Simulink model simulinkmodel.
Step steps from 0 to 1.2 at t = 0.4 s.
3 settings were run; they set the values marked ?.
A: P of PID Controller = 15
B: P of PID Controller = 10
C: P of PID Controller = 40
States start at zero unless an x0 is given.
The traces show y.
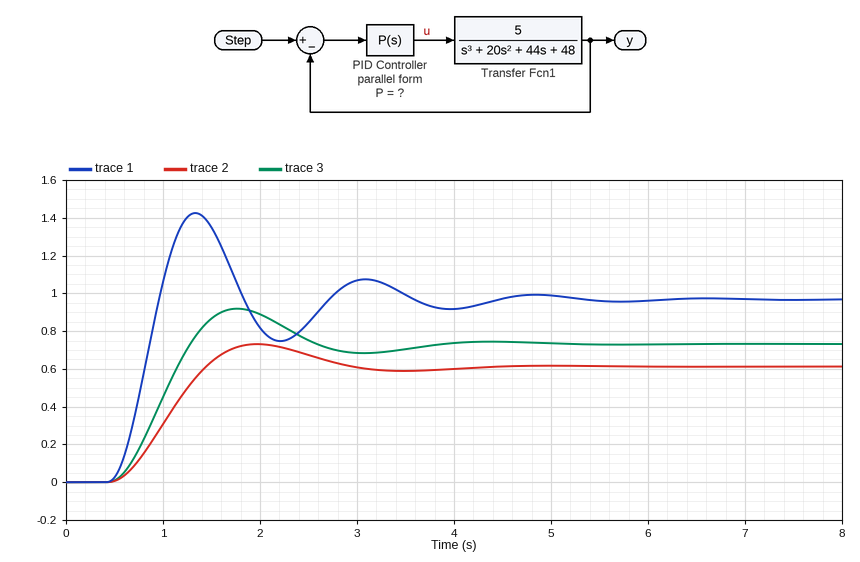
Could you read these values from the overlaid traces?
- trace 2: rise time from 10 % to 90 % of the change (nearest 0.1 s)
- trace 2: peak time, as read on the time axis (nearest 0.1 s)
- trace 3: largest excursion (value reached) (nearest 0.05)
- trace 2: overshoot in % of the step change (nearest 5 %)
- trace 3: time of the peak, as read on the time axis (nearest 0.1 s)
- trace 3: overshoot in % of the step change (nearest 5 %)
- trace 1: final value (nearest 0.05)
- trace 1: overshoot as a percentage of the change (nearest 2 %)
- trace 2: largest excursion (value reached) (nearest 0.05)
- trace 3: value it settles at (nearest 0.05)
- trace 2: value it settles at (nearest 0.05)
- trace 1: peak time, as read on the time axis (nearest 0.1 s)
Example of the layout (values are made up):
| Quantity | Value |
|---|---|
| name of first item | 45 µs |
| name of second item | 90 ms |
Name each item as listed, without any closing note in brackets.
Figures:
| Quantity | Value |
|---|---|
| trace 2: rise time from 10 % to 90 % of the change | 0.7 s |
| trace 2: peak time, as read on the time axis | 2.0 s |
| trace 3: largest excursion (value reached) | 0.90 |
| trace 2: overshoot in % of the step change | 20 % |
| trace 3: time of the peak, as read on the time axis | 1.8 s |
| trace 3: overshoot in % of the step change | 25 % |
| trace 1: final value | 0.95 |
| trace 1: overshoot as a percentage of the change | 48 % |
| trace 2: largest excursion (value reached) | 0.75 |
| trace 3: value it settles at | 0.75 |
| trace 2: value it settles at | 0.60 |
| trace 1: peak time, as read on the time axis | 1.3 s |
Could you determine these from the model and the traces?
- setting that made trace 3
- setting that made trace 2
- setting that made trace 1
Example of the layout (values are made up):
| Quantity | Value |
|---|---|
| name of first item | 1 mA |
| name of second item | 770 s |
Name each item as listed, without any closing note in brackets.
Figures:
| Quantity | Value |
|---|---|
| setting that made trace 3 | A |
| setting that made trace 2 | B |
| setting that made trace 1 | C |
